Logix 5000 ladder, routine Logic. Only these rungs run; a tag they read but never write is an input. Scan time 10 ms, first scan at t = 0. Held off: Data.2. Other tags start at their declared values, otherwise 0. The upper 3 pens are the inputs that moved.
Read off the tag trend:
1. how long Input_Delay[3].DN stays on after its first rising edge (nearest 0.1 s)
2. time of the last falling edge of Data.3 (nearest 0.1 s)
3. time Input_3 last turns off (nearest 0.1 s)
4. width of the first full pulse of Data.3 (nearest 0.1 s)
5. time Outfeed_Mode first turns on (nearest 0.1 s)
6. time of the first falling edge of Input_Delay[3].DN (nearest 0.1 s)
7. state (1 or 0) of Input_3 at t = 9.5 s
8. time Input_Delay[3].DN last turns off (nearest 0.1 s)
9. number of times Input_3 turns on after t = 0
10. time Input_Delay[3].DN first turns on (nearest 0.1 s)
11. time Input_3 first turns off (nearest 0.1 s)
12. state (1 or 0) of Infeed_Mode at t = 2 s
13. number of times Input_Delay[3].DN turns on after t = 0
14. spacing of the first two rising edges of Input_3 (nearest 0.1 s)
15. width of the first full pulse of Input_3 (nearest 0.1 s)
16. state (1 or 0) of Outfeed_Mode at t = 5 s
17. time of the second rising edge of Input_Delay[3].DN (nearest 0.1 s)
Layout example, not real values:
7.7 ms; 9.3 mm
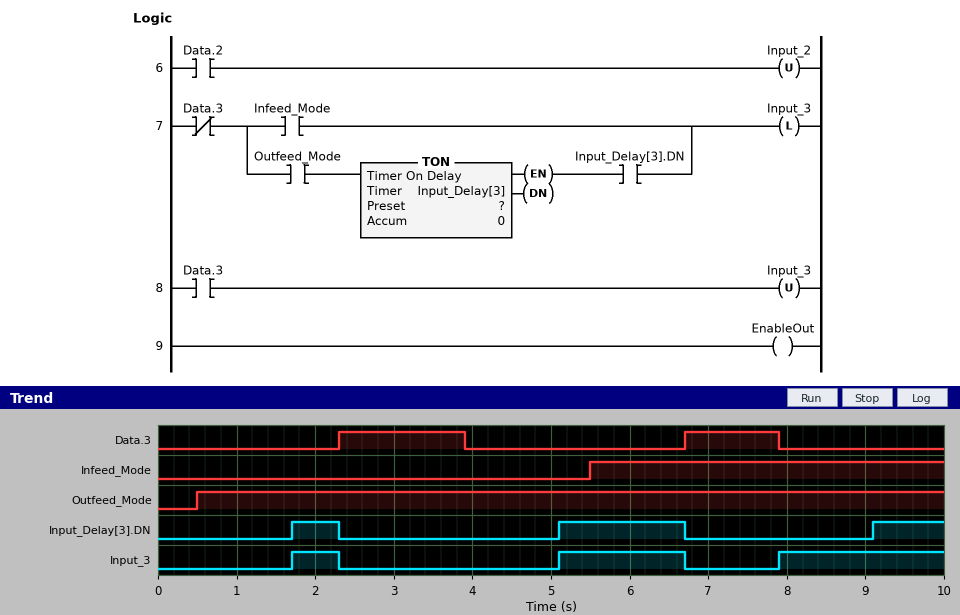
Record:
0.6 s; 7.9 s; 6.7 s; 1.6 s; 0.5 s; 2.3 s; 1; 6.7 s; 3; 1.7 s; 2.3 s; 0; 3; 3.4 s; 0.6 s; 1; 5.1 s
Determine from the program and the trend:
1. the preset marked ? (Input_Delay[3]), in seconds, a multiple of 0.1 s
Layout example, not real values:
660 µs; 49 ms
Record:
1.2 s
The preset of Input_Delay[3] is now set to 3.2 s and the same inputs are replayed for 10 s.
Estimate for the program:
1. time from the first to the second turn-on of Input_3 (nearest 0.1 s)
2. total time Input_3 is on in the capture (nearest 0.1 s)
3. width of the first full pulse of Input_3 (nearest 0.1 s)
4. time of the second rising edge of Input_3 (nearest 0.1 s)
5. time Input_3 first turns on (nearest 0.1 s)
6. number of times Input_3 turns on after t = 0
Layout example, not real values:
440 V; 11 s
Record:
2.4 s; 3.3 s; 1.2 s; 7.9 s; 5.5 s; 2
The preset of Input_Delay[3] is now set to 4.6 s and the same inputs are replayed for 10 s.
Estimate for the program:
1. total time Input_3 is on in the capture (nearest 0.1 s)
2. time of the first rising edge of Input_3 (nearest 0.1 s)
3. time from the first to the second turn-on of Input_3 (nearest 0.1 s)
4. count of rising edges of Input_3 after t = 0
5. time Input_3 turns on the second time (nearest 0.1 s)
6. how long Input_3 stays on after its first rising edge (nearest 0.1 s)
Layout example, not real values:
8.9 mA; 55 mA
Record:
3.3 s; 5.5 s; 2.4 s; 2; 7.9 s; 1.2 s
